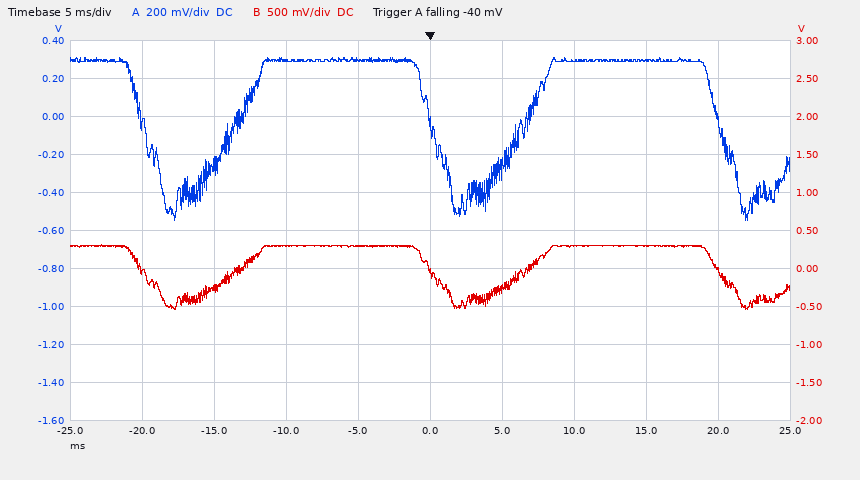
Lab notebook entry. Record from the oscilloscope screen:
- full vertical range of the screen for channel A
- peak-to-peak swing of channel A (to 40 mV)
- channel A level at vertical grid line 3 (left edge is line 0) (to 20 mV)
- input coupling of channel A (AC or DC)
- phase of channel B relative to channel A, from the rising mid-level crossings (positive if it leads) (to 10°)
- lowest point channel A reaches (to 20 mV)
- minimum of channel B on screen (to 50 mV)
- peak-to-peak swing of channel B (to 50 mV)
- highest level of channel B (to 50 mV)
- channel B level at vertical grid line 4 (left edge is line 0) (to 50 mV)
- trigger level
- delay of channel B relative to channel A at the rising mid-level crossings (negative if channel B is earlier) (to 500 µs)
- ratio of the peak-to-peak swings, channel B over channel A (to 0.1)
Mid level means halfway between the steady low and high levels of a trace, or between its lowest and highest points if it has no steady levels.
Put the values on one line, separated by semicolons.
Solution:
2 V; 840 mV; 300 mV; DC; 0°; -540 mV; -550 mV; 850 mV; 300 mV; 300 mV; -40 mV; 0.0 ms; 1.0
